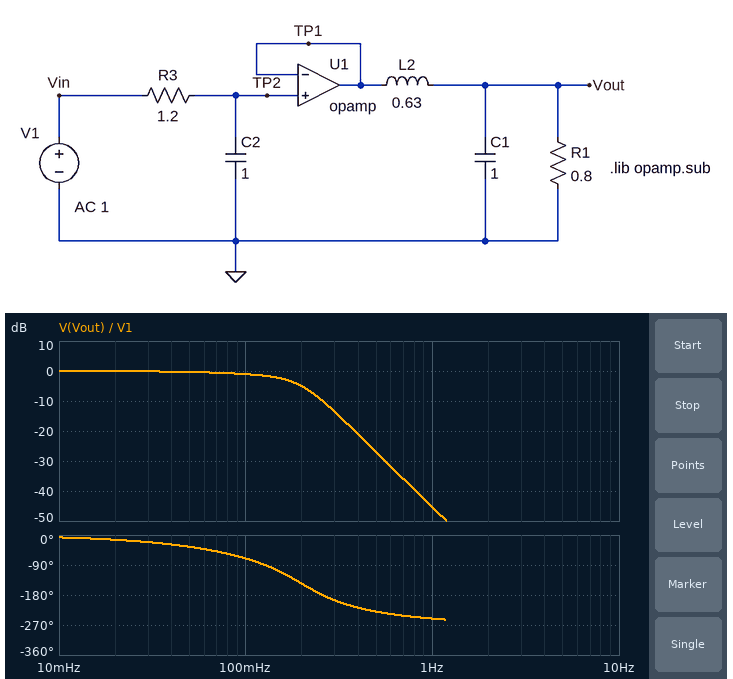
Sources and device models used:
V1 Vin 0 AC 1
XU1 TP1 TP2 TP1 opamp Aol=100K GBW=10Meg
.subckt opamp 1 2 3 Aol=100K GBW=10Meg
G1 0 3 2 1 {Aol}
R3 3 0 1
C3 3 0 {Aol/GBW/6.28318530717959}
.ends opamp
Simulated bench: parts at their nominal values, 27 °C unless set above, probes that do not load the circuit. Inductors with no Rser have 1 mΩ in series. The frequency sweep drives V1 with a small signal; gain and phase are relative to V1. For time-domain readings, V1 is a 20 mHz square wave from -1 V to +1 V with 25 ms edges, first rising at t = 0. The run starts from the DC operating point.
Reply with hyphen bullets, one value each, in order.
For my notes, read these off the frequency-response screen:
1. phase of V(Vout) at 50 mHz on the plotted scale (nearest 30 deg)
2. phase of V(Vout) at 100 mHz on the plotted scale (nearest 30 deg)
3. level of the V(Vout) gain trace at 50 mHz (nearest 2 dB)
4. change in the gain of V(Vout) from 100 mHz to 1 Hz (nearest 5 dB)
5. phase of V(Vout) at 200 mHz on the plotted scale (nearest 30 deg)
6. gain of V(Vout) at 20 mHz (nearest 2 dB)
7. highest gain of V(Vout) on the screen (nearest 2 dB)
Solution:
- -30 deg
- -60 deg
- 0 dB
- -45 dB
- -150 deg
- 0 dB
- 0 dB
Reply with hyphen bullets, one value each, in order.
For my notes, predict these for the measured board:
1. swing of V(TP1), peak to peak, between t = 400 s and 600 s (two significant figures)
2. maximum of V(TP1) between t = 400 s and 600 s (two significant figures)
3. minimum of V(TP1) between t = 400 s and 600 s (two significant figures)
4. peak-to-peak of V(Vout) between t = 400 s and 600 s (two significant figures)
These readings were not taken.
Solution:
- 2.0 V
- 1.0 V
- -1.0 V
- 2.1 V
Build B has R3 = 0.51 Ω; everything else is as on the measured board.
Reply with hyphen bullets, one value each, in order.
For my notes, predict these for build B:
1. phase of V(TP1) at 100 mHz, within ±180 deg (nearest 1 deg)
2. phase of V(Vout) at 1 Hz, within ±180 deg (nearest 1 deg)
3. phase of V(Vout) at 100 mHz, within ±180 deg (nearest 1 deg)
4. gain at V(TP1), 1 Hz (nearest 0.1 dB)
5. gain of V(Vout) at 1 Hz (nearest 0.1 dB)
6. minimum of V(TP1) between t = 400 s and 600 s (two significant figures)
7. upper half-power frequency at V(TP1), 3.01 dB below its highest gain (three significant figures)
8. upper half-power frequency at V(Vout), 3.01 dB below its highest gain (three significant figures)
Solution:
- -18 deg
- 119 deg
- -51 deg
- -10.5 dB
- -38.3 dB
- -1.0 V
- 312 mHz
- 217 mHz
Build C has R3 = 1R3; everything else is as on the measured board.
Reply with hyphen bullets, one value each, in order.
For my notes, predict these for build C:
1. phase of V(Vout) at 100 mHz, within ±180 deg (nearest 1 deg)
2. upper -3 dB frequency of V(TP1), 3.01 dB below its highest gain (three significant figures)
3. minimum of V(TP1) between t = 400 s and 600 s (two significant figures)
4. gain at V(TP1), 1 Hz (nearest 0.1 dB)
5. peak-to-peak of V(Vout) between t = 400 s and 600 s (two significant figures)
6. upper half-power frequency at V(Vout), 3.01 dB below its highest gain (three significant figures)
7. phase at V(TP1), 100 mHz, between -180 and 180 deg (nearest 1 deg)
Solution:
- -73 deg
- 122 mHz
- -1.0 V
- -18.3 dB
- 2.0 V
- 157 mHz
- -39 deg
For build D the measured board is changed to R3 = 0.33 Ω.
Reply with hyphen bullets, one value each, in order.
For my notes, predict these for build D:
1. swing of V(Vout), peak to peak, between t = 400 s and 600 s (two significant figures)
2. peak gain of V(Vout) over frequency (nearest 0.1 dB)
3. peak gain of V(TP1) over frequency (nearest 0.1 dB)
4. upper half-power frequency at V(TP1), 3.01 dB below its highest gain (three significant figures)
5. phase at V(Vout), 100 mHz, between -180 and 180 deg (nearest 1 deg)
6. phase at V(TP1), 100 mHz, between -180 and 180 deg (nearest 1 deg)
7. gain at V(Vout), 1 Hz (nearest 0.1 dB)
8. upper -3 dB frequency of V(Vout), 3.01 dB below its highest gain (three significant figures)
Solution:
- 2.6 V
- 0.9 dB
- 0 dB
- 482 mHz
- -45 deg
- -12 deg
- -35.0 dB
- 226 mHz
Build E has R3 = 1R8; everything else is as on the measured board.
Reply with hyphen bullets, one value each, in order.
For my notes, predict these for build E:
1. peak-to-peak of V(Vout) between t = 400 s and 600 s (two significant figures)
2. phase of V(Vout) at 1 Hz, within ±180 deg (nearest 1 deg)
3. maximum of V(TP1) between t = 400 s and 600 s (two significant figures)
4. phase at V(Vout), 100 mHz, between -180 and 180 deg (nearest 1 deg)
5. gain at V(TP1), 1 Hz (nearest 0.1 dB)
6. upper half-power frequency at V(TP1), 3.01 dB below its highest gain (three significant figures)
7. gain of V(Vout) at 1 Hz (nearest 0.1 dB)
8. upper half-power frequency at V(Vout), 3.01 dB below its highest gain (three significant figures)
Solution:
- 2.0 V
- 107 deg
- 1.0 V
- -82 deg
- -21.1 dB
- 88.4 mHz
- -48.8 dB
- 110 mHz
